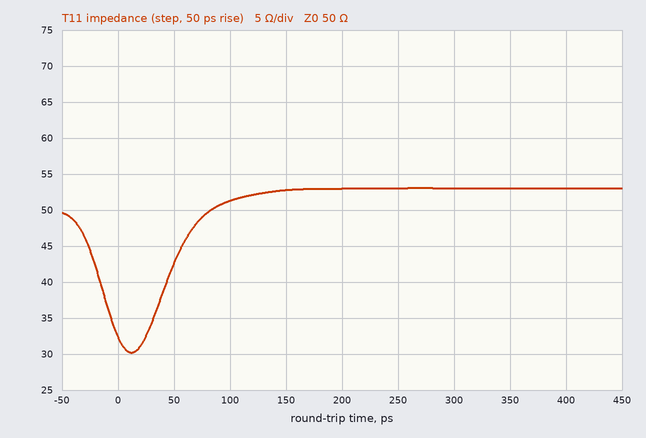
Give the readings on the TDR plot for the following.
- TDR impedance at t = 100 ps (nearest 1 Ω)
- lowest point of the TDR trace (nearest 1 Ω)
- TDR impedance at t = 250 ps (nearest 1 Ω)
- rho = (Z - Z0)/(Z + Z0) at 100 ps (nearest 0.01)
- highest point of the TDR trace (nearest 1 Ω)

51 Ω
30 Ω
53 Ω
+0.01
53 Ω
